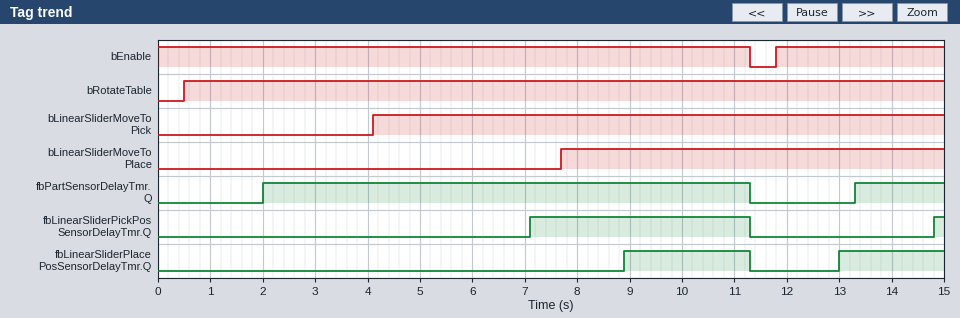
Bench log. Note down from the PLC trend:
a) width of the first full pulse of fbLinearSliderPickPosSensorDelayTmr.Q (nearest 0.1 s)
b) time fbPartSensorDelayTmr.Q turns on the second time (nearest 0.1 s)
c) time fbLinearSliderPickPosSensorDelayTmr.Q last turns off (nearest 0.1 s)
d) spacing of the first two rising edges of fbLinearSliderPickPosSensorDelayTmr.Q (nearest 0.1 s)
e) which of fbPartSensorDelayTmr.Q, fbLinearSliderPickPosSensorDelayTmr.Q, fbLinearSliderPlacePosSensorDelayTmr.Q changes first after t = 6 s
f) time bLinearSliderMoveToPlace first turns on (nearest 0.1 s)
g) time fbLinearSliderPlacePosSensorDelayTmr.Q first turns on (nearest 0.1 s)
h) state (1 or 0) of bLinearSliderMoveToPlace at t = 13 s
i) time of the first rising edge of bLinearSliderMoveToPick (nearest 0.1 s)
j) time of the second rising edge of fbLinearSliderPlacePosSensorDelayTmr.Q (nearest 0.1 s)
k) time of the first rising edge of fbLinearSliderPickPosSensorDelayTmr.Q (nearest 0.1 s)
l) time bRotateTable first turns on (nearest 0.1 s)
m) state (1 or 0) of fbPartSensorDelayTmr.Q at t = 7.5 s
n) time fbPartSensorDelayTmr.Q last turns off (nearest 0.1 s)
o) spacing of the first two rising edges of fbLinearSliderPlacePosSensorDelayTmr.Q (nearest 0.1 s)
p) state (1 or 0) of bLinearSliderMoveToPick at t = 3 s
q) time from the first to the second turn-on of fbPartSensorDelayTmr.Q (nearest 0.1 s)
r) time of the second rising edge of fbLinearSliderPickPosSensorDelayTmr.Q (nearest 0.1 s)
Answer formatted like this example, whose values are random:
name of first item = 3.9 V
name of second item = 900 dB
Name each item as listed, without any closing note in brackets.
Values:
width of the first full pulse of fbLinearSliderPickPosSensorDelayTmr.Q = 4.2 s
time fbPartSensorDelayTmr.Q turns on the second time = 13.3 s
time fbLinearSliderPickPosSensorDelayTmr.Q last turns off = 11.3 s
spacing of the first two rising edges of fbLinearSliderPickPosSensorDelayTmr.Q = 7.7 s
which of fbPartSensorDelayTmr.Q, fbLinearSliderPickPosSensorDelayTmr.Q, fbLinearSliderPlacePosSensorDelayTmr.Q changes first after t = 6 s = fbLinearSliderPickPosSensorDelayTmr.Q
time bLinearSliderMoveToPlace first turns on = 7.7 s
time fbLinearSliderPlacePosSensorDelayTmr.Q first turns on = 8.9 s
state (1 or 0) of bLinearSliderMoveToPlace at t = 13 s = 1
time of the first rising edge of bLinearSliderMoveToPick = 4.1 s
time of the second rising edge of fbLinearSliderPlacePosSensorDelayTmr.Q = 13.0 s
time of the first rising edge of fbLinearSliderPickPosSensorDelayTmr.Q = 7.1 s
time bRotateTable first turns on = 0.5 s
state (1 or 0) of fbPartSensorDelayTmr.Q at t = 7.5 s = 1
time fbPartSensorDelayTmr.Q last turns off = 11.3 s
spacing of the first two rising edges of fbLinearSliderPlacePosSensorDelayTmr.Q = 4.1 s
state (1 or 0) of bLinearSliderMoveToPick at t = 3 s = 0
time from the first to the second turn-on of fbPartSensorDelayTmr.Q = 11.3 s
time of the second rising edge of fbLinearSliderPickPosSensorDelayTmr.Q = 14.8 s
